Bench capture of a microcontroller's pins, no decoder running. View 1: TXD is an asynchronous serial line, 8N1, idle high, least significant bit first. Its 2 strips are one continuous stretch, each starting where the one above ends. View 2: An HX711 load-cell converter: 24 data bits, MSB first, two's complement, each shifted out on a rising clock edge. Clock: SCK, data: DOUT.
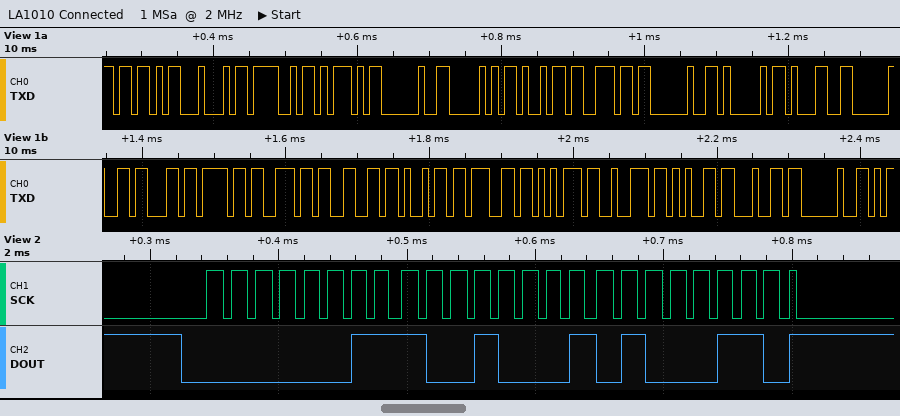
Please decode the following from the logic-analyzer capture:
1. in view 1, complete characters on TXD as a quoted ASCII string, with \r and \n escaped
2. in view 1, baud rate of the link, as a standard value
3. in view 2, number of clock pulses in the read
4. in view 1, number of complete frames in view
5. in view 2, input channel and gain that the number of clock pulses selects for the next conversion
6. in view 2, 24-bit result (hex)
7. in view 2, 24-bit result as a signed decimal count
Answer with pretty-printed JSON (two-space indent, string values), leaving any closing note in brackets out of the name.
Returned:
{
  "in view 1, complete characters on TXD as a quoted ASCII string, with \\r and \\n escaped": "\"[DO] Pin A1 configured \"",
  "in view 1, baud rate of the link, as a standard value": "115200 baud",
  "in view 2, number of clock pulses in the read": "25",
  "in view 1, number of complete frames in view": "23",
  "in view 2, input channel and gain that the number of clock pulses selects for the next conversion": "channel A, gain 128",
  "in view 2, 24-bit result": "0x039146",
  "in view 2, 24-bit result as a signed decimal count": "233798"
}
